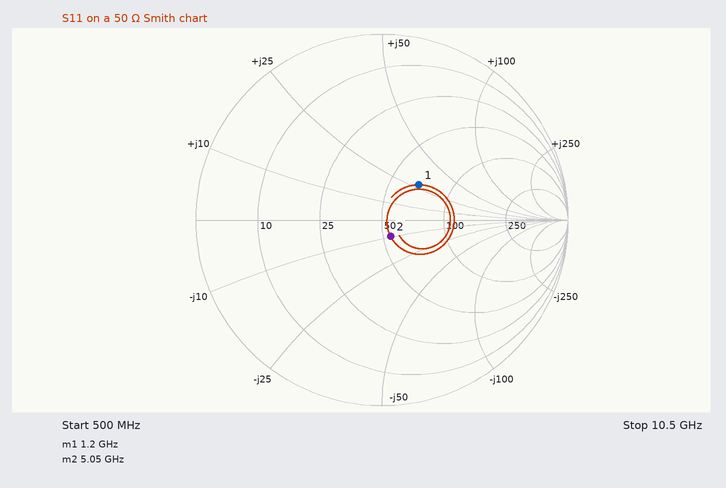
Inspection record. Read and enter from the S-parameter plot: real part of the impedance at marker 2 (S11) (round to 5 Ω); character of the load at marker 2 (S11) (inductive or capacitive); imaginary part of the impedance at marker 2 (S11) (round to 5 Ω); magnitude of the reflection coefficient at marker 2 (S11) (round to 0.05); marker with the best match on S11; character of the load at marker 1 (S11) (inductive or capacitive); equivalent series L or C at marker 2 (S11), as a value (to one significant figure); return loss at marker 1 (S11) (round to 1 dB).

55 Ω
capacitive
-10 Ω
0.10
marker 2
inductive
3 pF
11 dB
